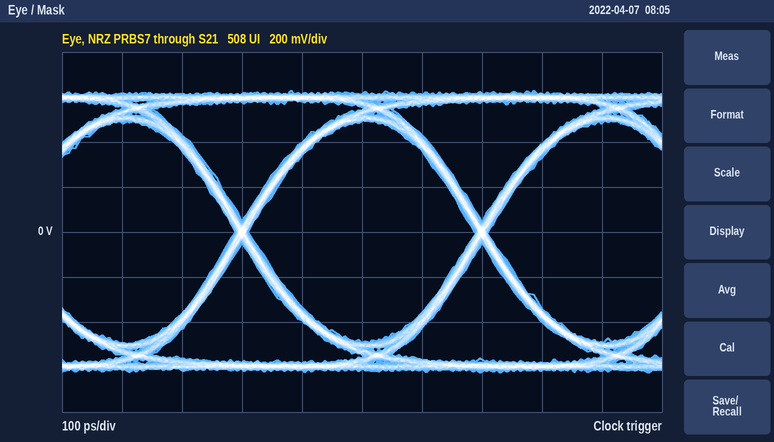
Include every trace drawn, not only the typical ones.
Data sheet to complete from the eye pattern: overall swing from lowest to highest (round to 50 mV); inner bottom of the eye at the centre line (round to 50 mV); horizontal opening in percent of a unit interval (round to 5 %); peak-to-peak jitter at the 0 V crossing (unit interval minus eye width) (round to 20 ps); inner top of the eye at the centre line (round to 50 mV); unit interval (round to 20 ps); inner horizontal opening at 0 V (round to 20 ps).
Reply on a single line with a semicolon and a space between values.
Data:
1.25 V; -500 mV; 95 %; 20 ps; 500 mV; 400 ps; 380 ps
